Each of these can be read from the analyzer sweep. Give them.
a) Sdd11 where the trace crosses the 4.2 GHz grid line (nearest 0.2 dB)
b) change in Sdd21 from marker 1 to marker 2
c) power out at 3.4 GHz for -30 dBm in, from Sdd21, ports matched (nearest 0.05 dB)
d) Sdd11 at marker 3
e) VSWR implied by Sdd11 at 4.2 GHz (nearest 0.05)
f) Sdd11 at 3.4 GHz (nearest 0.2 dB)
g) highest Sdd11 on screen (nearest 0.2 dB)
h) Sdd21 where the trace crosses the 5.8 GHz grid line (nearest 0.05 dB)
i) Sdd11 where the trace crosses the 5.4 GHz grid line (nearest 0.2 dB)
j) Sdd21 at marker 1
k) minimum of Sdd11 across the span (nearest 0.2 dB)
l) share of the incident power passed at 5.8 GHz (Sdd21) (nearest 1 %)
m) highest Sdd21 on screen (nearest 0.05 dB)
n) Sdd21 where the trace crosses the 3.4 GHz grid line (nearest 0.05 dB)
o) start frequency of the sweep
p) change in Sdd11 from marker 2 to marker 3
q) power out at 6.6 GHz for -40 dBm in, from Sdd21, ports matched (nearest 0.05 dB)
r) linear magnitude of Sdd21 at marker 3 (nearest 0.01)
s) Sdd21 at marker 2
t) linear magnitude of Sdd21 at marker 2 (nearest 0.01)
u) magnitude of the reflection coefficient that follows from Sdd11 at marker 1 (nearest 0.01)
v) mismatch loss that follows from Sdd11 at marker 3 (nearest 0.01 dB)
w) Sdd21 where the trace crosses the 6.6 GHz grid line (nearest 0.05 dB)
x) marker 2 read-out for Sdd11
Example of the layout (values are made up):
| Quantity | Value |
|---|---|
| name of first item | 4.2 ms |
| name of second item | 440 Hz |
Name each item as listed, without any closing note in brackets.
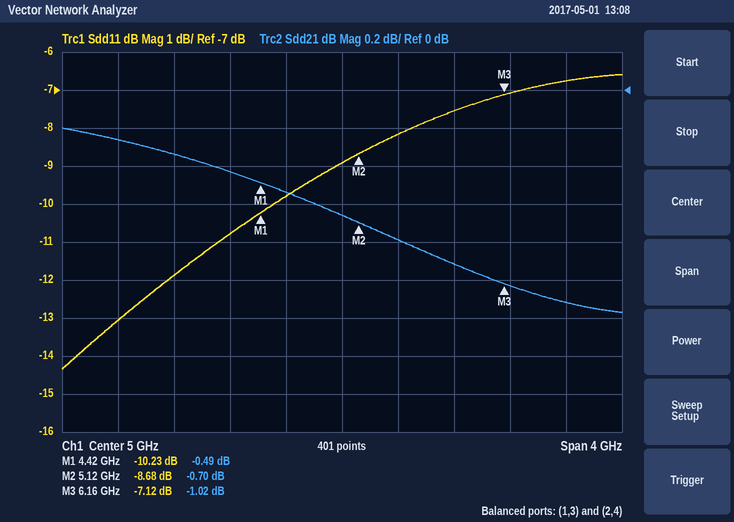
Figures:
| Quantity | Value |
|---|---|
| Sdd11 where the trace crosses the 4.2 GHz grid line | -10.8 dB |
| change in Sdd21 from marker 1 to marker 2 | -0.21 dB |
| power out at 3.4 GHz for -30 dBm in, from Sdd21, ports matched | -30.25 dBm |
| Sdd11 at marker 3 | -7.12 dB |
| VSWR implied by Sdd11 at 4.2 GHz | 1.80 |
| Sdd11 at 3.4 GHz | -13.0 dB |
| highest Sdd11 on screen | -6.6 dB |
| Sdd21 where the trace crosses the 5.8 GHz grid line | -0.90 dB |
| Sdd11 where the trace crosses the 5.4 GHz grid line | -8.2 dB |
| Sdd21 at marker 1 | -0.49 dB |
| minimum of Sdd11 across the span | -14.4 dB |
| share of the incident power passed at 5.8 GHz (Sdd21) | 81 % |
| highest Sdd21 on screen | -0.20 dB |
| Sdd21 where the trace crosses the 3.4 GHz grid line | -0.25 dB |
| start frequency of the sweep | 3 GHz |
| change in Sdd11 from marker 2 to marker 3 | 1.56 dB |
| power out at 6.6 GHz for -40 dBm in, from Sdd21, ports matched | -41.10 dBm |
| linear magnitude of Sdd21 at marker 3 | 0.89 |
| Sdd21 at marker 2 | -0.70 dB |
| linear magnitude of Sdd21 at marker 2 | 0.92 |
| magnitude of the reflection coefficient that follows from Sdd11 at marker 1 | 0.31 |
| mismatch loss that follows from Sdd11 at marker 3 | 0.94 dB |
| Sdd21 where the trace crosses the 6.6 GHz grid line | -1.10 dB |
| marker 2 read-out for Sdd11 | -8.68 dB |
